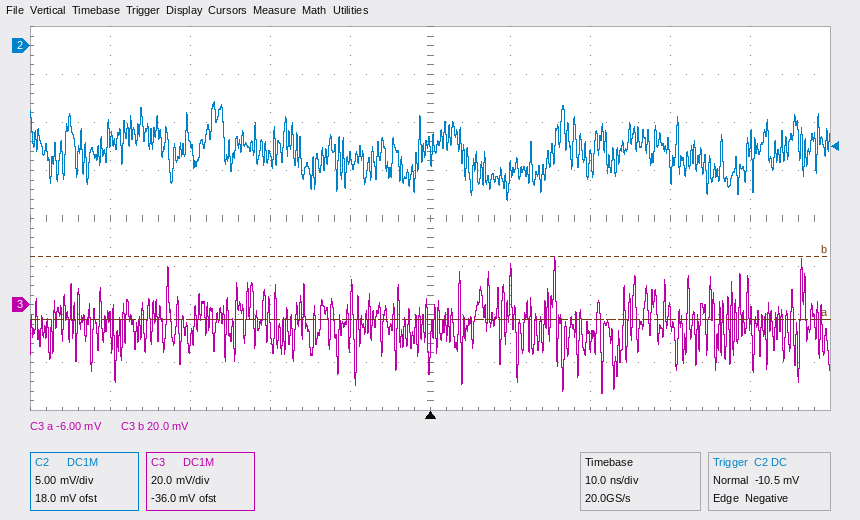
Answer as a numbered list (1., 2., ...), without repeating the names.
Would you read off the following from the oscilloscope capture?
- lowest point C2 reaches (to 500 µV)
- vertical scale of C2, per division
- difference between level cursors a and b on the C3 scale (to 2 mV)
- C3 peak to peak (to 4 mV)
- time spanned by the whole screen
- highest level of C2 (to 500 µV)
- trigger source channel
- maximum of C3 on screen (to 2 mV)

1. -16.0 mV
2. 5 mV
3. 26 mV
4. 56 mV
5. 100 ns
6. -6.0 mV
7. C2
8. 20 mV
